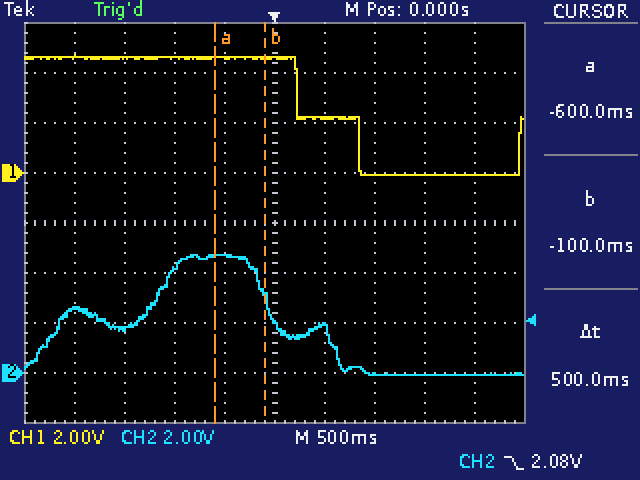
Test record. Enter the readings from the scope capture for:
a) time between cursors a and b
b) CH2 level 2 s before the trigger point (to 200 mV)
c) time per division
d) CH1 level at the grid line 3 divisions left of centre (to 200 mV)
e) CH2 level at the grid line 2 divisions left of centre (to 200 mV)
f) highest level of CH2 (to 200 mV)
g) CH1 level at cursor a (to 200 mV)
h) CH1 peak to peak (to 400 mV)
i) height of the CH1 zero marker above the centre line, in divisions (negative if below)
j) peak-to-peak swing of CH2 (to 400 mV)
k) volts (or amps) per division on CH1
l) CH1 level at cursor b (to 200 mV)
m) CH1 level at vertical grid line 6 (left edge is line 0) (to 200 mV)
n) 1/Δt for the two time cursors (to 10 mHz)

500 ms
2.6 V
500 ms
4.6 V
4.2 V
4.8 V
4.6 V
4.8 V
+1.0 div
4.8 V
2 V
4.6 V
2.2 V
2.00 Hz
